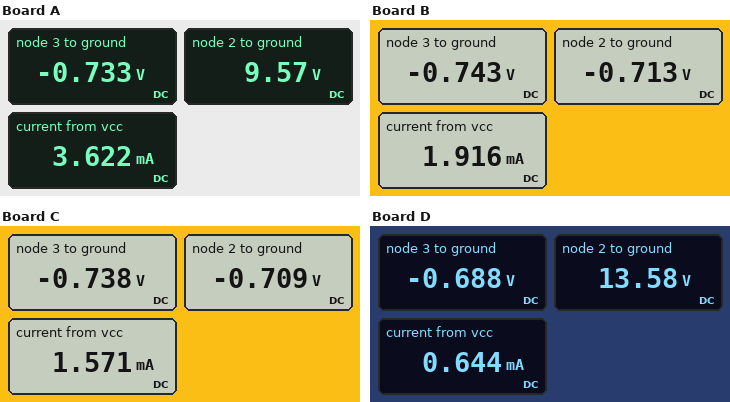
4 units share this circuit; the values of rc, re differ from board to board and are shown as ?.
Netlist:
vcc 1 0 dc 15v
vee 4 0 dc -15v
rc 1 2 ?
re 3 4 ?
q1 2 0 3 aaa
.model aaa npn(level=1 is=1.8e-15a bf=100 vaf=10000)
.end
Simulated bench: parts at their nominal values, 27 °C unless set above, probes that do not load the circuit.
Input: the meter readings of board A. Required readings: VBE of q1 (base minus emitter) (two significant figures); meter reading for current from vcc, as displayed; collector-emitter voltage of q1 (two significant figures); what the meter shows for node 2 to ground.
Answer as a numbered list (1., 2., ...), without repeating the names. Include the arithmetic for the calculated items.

1. 0 V - (-733 mV) = 730 mV
2. 3.622 mA
3. 9.57 V - (-733 mV) = 10 V
4. 9.57 V
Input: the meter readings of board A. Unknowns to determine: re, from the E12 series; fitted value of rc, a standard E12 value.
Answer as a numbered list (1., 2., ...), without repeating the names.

1. 3.9 kΩ
2. 1.5 kΩ
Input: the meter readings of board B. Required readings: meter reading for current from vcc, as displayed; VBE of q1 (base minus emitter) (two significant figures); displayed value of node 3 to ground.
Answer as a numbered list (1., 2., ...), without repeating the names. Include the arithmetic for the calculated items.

1. 1.916 mA
2. 0 V - (-743 mV) = 740 mV
3. -0.743 V
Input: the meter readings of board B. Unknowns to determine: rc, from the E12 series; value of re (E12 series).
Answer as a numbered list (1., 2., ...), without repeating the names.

1. 8.2 kΩ
2. 3.9 kΩ
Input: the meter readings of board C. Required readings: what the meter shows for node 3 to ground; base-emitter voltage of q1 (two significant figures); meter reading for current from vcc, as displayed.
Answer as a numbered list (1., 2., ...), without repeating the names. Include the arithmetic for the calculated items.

1. -0.738 V
2. 0 V - (-738 mV) = 740 mV
3. 1.571 mA
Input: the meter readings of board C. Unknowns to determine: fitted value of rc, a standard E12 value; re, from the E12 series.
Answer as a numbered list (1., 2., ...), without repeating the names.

1. 10 kΩ
2. 4.7 kΩ
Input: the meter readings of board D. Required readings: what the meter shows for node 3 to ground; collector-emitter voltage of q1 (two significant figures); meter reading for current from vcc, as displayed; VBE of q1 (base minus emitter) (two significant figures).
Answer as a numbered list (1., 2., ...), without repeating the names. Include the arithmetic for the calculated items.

1. -0.688 V
2. 13.58 V - (-688 mV) = 14 V
3. 0.644 mA
4. 0 V - (-688 mV) = 690 mV
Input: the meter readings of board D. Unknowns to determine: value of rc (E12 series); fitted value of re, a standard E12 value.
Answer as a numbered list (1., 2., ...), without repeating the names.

1. 2.2 kΩ
2. 22 kΩ
